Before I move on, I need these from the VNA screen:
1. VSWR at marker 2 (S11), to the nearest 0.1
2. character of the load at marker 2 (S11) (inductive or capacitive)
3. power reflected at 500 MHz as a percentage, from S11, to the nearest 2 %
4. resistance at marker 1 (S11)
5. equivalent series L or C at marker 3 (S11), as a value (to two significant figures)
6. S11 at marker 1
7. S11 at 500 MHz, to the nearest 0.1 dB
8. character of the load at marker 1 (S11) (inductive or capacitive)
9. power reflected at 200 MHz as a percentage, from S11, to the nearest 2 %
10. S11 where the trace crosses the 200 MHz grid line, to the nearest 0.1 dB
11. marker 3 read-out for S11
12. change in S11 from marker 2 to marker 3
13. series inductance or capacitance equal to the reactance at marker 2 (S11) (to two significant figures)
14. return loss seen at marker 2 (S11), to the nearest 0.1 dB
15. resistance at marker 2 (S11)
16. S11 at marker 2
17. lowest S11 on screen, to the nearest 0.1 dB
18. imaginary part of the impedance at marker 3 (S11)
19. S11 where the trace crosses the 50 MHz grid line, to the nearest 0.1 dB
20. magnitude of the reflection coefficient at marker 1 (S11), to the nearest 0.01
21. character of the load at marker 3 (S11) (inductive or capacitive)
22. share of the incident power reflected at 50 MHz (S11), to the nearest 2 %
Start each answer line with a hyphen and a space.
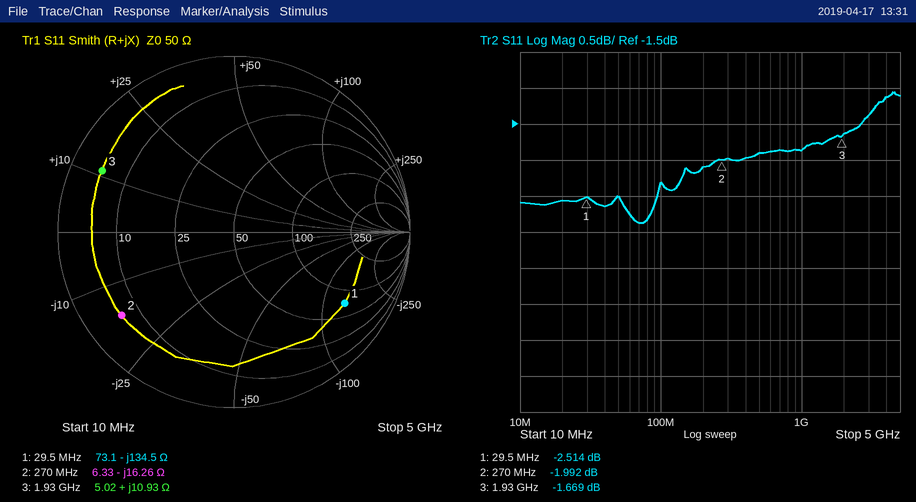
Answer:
- 8.8
- capacitive
- 64 %
- 73.1 Ω
- 900 pH
- -2.514 dB
- -1.9 dB
- capacitive
- 62 %
- -2.1 dB
- -1.669 dB
- 0.323 dB
- 36 pF
- 2.0 dB
- 6.33 Ω
- -1.992 dB
- -2.9 dB
- +10.93 Ω
- -2.5 dB
- 0.75
- inductive
- 56 %
